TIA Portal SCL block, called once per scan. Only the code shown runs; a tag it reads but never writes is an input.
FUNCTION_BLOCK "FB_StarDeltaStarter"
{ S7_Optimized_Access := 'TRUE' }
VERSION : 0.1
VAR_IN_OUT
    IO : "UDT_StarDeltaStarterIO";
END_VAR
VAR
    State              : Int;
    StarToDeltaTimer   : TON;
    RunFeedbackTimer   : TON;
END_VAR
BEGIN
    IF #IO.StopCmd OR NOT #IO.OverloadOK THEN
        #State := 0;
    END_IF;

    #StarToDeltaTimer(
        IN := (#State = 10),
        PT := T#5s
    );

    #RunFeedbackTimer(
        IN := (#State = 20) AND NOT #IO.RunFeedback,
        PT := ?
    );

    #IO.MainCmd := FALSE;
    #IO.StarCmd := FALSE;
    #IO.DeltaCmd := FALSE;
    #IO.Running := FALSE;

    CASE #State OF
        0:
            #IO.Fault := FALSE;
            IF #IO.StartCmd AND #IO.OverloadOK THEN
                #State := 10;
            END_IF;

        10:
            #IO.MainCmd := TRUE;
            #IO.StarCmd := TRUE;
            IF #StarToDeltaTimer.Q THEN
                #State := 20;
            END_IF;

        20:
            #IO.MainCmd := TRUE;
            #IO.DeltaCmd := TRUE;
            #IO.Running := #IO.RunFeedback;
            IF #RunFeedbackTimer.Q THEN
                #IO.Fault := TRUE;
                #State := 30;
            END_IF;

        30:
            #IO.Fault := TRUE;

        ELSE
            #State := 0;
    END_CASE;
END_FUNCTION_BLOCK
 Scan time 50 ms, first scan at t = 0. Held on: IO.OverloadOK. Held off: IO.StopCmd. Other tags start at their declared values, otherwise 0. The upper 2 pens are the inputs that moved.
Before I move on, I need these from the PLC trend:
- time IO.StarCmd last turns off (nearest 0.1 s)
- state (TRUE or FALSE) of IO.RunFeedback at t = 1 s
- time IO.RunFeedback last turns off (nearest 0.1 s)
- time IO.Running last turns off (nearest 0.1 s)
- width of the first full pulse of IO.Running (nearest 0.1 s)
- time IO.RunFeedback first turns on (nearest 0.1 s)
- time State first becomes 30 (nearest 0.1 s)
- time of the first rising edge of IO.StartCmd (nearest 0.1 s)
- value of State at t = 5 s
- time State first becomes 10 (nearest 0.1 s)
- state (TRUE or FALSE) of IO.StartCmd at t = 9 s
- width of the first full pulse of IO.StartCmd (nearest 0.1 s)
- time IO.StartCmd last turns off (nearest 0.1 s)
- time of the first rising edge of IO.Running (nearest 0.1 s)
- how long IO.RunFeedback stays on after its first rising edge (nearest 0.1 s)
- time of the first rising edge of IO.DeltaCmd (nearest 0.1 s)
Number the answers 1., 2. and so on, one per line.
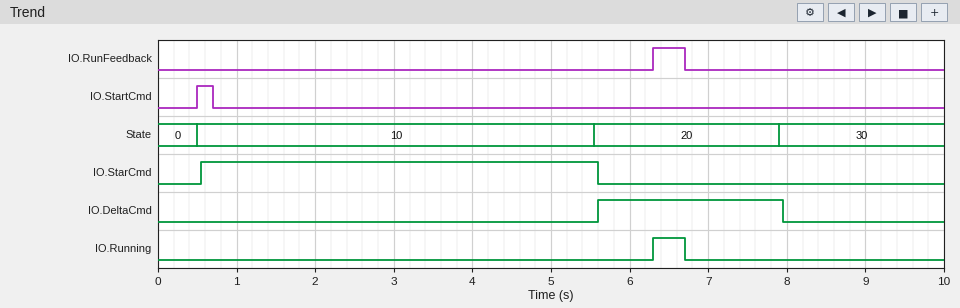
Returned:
1. 5.6 s
2. FALSE
3. 6.7 s
4. 6.7 s
5. 0.4 s
6. 6.3 s
7. 7.9 s
8. 0.5 s
9. 10
10. 0.5 s
11. FALSE
12. 0.2 s
13. 0.7 s
14. 6.3 s
15. 0.4 s
16. 5.6 s
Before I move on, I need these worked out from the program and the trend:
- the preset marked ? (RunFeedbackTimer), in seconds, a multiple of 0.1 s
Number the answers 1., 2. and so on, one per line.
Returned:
1. 1.2 s
